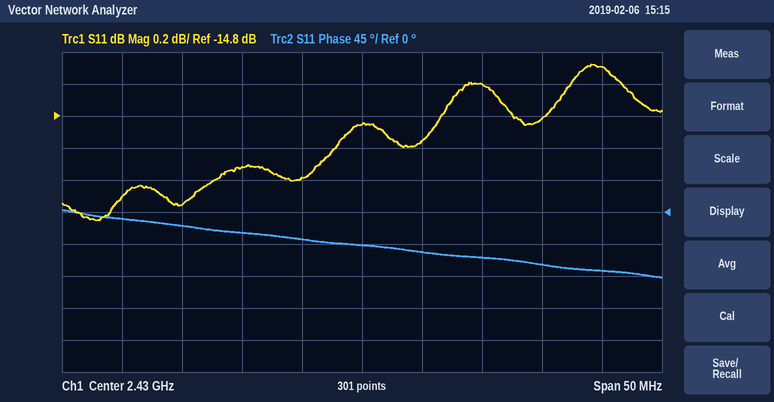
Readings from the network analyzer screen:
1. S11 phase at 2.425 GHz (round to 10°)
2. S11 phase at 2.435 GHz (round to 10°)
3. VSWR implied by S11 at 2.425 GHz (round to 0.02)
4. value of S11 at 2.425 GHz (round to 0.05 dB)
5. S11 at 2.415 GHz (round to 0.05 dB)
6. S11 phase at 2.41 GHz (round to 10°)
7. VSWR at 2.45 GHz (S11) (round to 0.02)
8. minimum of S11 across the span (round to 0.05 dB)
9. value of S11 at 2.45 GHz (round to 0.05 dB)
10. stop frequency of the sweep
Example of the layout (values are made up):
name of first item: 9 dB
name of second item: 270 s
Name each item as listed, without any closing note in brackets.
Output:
S11 phase at 2.425 GHz: -40°
S11 phase at 2.435 GHz: -60°
VSWR implied by S11 at 2.425 GHz: 1.42
value of S11 at 2.425 GHz: -15.20 dB
S11 at 2.415 GHz: -15.35 dB
S11 phase at 2.41 GHz: -10°
VSWR at 2.45 GHz (S11): 1.46
minimum of S11 across the span: -15.45 dB
value of S11 at 2.45 GHz: -14.50 dB
stop frequency of the sweep: 2.455 GHz
